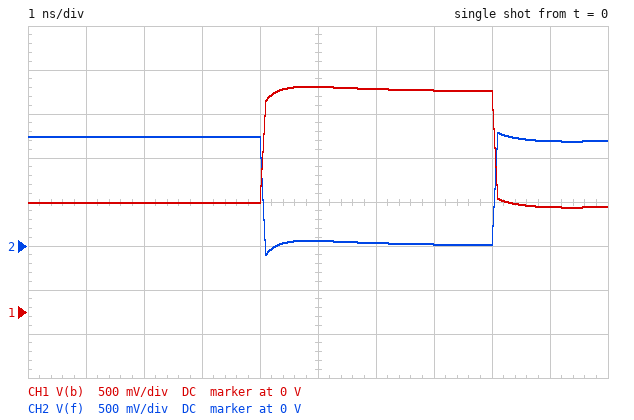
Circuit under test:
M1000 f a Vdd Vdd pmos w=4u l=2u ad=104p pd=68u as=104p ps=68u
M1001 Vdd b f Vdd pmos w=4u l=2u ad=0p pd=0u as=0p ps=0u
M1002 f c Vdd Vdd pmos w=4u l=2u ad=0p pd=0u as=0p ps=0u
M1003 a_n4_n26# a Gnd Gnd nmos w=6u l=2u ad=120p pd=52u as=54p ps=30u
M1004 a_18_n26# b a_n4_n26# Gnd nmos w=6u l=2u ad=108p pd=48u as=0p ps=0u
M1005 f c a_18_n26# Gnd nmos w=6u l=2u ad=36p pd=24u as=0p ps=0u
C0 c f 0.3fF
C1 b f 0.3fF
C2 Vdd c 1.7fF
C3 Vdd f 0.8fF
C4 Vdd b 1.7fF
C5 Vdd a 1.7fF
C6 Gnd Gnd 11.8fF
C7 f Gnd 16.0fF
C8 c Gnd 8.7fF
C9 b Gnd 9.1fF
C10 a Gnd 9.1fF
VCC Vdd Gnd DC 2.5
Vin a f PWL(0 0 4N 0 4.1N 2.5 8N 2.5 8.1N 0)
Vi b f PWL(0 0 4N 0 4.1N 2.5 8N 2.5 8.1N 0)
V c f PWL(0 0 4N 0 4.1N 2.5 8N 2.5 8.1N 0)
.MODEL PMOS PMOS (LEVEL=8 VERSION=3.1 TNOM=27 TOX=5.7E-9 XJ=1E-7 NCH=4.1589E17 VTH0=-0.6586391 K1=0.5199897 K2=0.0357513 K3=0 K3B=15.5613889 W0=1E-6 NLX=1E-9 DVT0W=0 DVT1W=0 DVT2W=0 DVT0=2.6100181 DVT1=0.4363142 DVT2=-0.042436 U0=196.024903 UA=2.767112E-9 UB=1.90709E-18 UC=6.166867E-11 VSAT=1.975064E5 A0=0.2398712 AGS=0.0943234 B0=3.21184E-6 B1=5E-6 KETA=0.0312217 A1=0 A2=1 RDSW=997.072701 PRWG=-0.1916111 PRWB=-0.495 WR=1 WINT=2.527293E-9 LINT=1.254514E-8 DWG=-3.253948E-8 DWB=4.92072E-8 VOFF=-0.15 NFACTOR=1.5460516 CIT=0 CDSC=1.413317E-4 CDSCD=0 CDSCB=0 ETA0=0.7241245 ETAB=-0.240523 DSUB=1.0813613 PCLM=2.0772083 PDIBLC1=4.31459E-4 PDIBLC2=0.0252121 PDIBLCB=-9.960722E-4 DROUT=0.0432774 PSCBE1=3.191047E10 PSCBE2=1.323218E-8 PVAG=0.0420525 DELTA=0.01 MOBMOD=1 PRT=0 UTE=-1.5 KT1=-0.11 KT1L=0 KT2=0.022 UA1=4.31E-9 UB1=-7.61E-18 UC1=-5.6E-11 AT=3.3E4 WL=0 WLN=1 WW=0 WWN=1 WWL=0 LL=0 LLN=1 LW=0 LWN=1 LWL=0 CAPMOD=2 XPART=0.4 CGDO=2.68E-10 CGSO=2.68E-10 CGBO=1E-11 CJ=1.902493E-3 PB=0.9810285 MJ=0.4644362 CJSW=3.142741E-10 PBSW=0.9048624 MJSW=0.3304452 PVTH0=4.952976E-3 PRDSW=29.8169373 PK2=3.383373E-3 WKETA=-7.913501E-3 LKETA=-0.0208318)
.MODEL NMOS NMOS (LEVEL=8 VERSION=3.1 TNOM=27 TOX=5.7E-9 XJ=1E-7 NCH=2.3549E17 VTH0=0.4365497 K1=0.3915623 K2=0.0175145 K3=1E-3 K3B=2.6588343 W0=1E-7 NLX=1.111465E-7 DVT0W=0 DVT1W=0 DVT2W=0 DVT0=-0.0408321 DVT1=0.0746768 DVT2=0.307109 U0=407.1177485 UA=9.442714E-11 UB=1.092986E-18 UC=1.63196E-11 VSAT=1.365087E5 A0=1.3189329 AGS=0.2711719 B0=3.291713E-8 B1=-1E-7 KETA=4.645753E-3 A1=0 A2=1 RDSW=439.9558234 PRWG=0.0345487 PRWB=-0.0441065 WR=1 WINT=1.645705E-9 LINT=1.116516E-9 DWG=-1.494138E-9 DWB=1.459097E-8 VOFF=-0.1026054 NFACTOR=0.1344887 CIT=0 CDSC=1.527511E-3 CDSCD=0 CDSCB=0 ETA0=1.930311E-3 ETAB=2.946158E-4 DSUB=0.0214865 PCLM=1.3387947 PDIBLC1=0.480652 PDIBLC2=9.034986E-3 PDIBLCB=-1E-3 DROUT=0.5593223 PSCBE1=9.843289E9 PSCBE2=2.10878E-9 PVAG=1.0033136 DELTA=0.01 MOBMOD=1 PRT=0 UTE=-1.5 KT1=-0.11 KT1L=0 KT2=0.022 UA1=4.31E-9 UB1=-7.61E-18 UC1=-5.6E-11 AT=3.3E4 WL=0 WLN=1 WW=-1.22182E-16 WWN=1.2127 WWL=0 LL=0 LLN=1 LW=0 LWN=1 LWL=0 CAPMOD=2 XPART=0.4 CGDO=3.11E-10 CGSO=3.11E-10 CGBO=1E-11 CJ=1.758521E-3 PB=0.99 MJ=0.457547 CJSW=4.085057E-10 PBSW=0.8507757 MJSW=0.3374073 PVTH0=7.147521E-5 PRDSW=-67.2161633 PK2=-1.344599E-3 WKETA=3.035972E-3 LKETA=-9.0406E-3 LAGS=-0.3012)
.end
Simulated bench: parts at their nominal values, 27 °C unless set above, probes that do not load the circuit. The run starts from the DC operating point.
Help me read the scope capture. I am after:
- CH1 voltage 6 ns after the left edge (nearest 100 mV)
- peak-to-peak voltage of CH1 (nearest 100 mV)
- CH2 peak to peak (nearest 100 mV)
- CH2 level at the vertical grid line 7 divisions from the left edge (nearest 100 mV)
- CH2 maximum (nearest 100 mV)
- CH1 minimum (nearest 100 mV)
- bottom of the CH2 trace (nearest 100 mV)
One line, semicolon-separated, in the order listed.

2.5 V; 1.4 V; 1.4 V; 0 V; 1.3 V; 1.2 V; -100 mV
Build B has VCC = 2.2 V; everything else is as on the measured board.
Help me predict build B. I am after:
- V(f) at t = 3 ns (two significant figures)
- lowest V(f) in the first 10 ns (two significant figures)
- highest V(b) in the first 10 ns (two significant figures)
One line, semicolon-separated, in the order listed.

1.1 V; -240 mV; 2.5 V
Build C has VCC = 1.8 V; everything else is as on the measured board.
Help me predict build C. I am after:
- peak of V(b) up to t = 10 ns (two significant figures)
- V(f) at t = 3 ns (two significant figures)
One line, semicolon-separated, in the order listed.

2.5 V; 850 mV
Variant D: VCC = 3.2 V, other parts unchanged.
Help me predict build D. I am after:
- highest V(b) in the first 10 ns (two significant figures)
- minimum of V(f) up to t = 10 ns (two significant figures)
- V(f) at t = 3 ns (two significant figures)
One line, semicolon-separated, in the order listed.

2.8 V; 28 mV; 1.6 V
